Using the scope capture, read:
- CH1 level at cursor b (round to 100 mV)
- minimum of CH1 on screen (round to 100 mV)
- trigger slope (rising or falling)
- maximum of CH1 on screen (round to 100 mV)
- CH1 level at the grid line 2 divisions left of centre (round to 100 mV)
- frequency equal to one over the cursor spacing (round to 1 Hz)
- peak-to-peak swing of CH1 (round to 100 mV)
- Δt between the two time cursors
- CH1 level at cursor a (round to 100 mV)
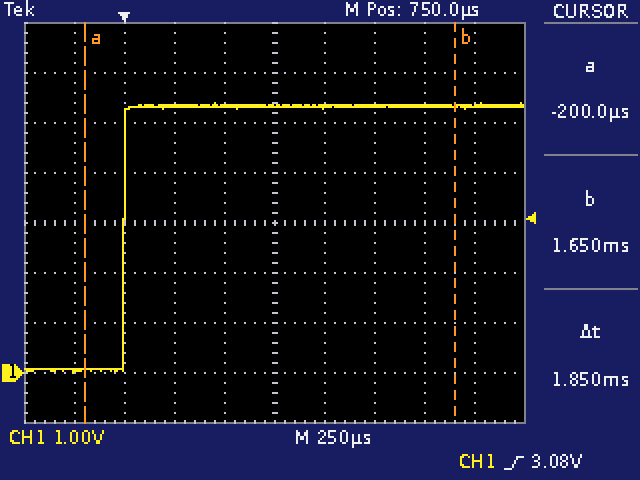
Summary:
5.3 V
0.0 V
rising
5.4 V
5.3 V
541 Hz
5.4 V
1.85 ms
100 mV
